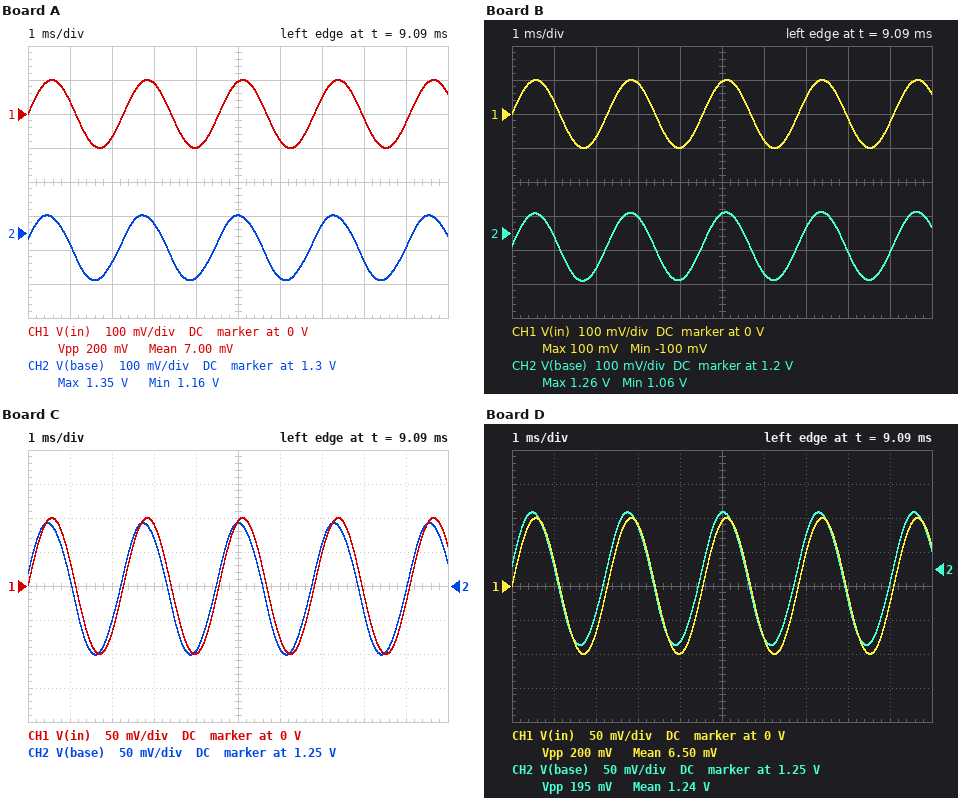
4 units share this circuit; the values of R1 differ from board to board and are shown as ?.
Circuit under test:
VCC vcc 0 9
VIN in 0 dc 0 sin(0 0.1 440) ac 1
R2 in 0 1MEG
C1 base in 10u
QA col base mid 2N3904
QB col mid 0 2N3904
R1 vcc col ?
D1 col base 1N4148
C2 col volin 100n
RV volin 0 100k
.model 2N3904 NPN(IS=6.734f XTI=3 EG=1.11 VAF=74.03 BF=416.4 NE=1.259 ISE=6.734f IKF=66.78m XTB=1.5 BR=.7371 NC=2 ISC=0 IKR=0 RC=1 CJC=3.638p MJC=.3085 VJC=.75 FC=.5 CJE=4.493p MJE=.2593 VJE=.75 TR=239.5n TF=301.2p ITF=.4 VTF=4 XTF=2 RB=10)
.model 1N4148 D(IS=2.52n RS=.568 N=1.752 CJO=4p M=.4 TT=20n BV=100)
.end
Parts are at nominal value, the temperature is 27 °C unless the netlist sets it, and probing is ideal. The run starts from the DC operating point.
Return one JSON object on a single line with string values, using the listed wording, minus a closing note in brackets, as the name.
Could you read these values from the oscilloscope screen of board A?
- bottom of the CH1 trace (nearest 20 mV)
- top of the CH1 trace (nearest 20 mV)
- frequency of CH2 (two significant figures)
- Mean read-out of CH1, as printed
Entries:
{"bottom of the CH1 trace": "-100 mV", "top of the CH1 trace": "100 mV", "frequency of CH2": "440 Hz", "Mean read-out of CH1, as printed": "7.00 mV"}
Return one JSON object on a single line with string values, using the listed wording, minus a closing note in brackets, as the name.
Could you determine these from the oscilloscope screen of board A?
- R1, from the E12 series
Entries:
{"R1, from the E12 series": "5.6 kΩ"}
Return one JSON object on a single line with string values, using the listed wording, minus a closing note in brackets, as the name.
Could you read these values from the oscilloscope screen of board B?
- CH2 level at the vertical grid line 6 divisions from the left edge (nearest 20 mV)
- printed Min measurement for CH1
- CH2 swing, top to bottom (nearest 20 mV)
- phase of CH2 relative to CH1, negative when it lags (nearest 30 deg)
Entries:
{"CH2 level at the vertical grid line 6 divisions from the left edge": "1.08 V", "printed Min measurement for CH1": "-100 mV", "CH2 swing, top to bottom": "200 mV", "phase of CH2 relative to CH1, negative when it lags": "0 deg"}
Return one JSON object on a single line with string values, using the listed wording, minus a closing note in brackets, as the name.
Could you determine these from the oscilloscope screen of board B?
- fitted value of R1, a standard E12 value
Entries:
{"fitted value of R1, a standard E12 value": "33 kΩ"}
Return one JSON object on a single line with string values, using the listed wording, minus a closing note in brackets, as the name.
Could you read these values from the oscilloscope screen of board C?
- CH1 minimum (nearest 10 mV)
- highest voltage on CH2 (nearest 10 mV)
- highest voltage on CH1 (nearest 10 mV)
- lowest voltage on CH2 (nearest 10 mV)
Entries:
{"CH1 minimum": "-100 mV", "highest voltage on CH2": "1.34 V", "highest voltage on CH1": "100 mV", "lowest voltage on CH2": "1.15 V"}
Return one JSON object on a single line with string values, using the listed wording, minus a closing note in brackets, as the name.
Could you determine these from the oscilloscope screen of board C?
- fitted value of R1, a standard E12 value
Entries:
{"fitted value of R1, a standard E12 value": "6.8 kΩ"}
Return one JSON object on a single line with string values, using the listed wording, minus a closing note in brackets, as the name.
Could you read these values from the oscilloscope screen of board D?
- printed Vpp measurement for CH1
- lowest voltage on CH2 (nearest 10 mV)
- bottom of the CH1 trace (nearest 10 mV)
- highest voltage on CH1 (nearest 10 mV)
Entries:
{"printed Vpp measurement for CH1": "200 mV", "lowest voltage on CH2": "1.14 V", "bottom of the CH1 trace": "-100 mV", "highest voltage on CH1": "100 mV"}
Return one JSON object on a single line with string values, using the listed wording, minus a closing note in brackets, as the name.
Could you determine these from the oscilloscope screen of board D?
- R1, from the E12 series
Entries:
{"R1, from the E12 series": "8.2 kΩ"}
